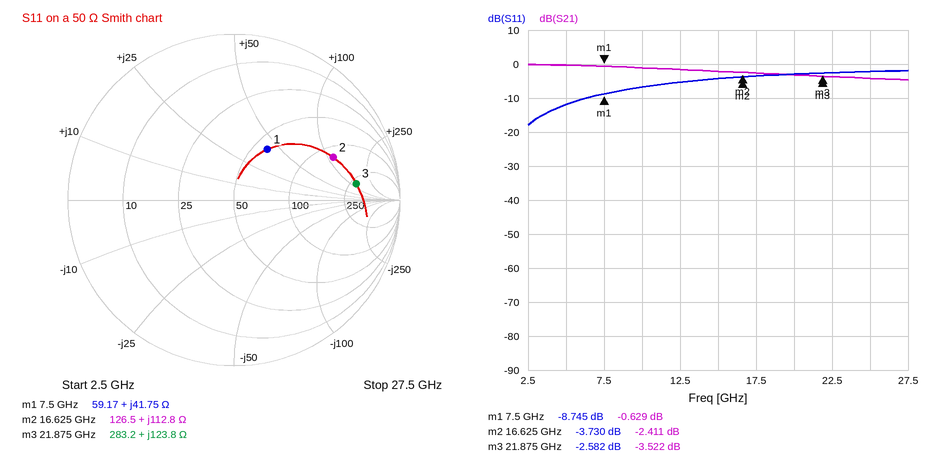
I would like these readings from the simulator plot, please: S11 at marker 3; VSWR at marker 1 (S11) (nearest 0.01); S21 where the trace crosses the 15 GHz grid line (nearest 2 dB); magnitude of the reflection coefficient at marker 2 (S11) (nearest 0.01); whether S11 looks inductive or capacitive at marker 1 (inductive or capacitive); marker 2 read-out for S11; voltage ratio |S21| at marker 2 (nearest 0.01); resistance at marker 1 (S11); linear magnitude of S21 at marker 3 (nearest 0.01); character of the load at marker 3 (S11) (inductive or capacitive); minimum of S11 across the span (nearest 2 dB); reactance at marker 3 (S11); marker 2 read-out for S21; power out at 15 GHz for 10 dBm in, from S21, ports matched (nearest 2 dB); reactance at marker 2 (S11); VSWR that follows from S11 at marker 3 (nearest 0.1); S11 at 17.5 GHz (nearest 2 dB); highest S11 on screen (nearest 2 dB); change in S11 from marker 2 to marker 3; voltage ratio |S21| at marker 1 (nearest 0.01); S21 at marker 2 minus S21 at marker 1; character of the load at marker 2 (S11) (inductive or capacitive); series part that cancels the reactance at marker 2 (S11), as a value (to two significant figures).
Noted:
-2.582 dB
2.15
-2 dB
0.65
inductive
-3.730 dB
0.76
59.17 Ω
0.67
inductive
-18 dB
+123.8 Ω
-2.411 dB
8 dBm
+112.8 Ω
6.8
-4 dB
-2 dB
1.148 dB
0.93
-1.782 dB
inductive
85 fF
